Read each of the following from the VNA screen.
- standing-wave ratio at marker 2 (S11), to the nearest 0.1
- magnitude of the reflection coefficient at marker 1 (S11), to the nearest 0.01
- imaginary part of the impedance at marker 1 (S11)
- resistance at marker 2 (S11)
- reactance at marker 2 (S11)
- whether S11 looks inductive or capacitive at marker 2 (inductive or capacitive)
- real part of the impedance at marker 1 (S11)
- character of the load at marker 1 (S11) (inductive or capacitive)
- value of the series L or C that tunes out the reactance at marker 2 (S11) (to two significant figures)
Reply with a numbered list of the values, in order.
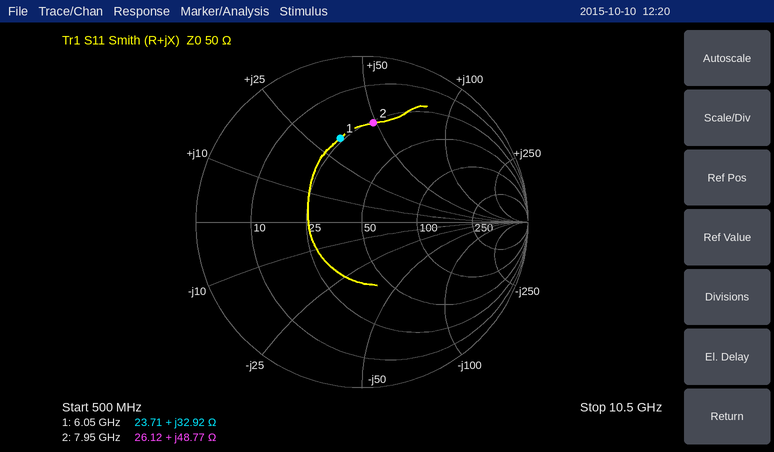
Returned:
1. 4.0
2. 0.52
3. +32.92 Ω
4. 26.12 Ω
5. +48.77 Ω
6. inductive
7. 23.71 Ω
8. inductive
9. 410 fF
